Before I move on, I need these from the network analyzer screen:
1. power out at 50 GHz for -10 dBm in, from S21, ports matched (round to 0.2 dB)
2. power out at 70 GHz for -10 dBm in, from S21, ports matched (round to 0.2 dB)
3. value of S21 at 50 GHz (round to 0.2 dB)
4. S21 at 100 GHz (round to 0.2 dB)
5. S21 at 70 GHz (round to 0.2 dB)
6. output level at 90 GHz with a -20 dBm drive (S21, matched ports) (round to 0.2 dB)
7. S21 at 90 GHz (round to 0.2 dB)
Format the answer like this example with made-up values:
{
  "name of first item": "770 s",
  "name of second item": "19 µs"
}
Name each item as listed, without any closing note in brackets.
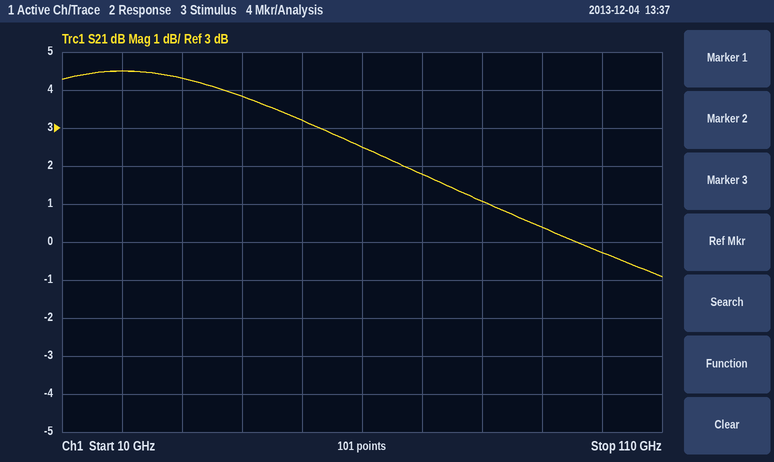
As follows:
{
  "power out at 50 GHz for -10 dBm in, from S21, ports matched": "-6.8 dBm",
  "power out at 70 GHz for -10 dBm in, from S21, ports matched": "-8.2 dBm",
  "value of S21 at 50 GHz": "3.2 dB",
  "S21 at 100 GHz": "-0.2 dB",
  "S21 at 70 GHz": "1.8 dB",
  "output level at 90 GHz with a -20 dBm drive (S21, matched ports)": "-19.6 dBm",
  "S21 at 90 GHz": "0.4 dB"
}
